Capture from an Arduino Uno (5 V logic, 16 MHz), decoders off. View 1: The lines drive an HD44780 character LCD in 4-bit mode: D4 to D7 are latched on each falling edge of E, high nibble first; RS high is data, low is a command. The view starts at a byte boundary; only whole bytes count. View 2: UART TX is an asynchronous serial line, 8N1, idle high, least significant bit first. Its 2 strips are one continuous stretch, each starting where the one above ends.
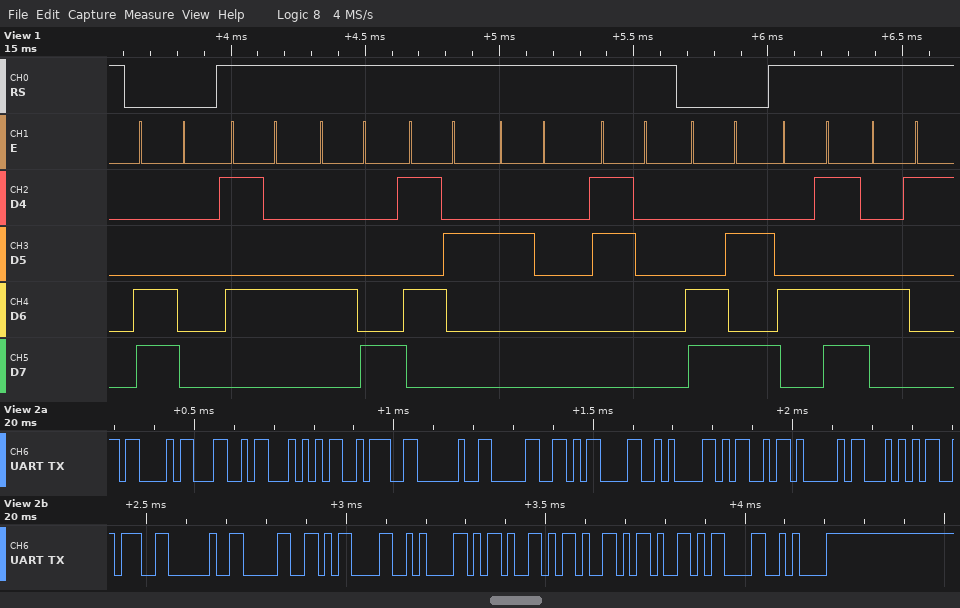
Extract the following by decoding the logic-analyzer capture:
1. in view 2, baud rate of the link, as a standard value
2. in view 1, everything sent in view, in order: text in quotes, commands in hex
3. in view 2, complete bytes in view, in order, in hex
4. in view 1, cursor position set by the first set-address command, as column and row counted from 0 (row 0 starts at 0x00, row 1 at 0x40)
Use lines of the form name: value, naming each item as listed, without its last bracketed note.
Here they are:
in view 2, baud rate of the link, as a standard value: 57600 baud
in view 1, everything sent in view, in order: text in quotes, commands in hex: 0xC0 "THR 0" 0xCA "MA"
in view 2, complete bytes in view, in order, in hex: 43 4C 54 3A 20 30 0D 0A 4D 41 54 3A 20 30 0D 0A 2D 2D 2D 0D 0A
in view 1, cursor position set by the first set-address command, as column and row counted from 0: column 0, row 1
